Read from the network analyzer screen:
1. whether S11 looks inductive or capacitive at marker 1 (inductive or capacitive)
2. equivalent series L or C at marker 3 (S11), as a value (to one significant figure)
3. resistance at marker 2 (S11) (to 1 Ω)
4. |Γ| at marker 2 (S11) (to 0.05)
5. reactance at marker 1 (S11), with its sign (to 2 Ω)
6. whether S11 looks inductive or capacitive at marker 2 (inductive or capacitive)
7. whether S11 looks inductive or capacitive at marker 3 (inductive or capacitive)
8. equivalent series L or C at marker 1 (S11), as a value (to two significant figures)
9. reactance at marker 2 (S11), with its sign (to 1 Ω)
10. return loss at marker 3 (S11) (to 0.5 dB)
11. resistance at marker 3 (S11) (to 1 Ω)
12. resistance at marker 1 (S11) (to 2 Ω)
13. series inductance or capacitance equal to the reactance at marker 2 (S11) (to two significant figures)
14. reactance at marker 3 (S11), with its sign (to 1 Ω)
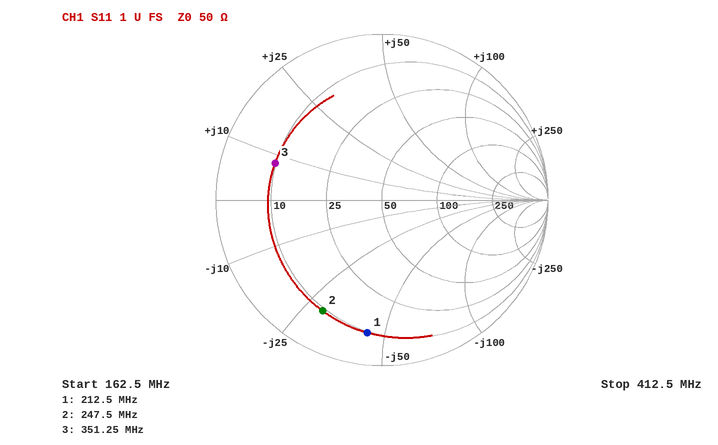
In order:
capacitive
4 nH
9 Ω
0.75
-44 Ω
capacitive
inductive
17 pF
-29 Ω
3.5 dB
10 Ω
10 Ω
22 pF
+8 Ω
